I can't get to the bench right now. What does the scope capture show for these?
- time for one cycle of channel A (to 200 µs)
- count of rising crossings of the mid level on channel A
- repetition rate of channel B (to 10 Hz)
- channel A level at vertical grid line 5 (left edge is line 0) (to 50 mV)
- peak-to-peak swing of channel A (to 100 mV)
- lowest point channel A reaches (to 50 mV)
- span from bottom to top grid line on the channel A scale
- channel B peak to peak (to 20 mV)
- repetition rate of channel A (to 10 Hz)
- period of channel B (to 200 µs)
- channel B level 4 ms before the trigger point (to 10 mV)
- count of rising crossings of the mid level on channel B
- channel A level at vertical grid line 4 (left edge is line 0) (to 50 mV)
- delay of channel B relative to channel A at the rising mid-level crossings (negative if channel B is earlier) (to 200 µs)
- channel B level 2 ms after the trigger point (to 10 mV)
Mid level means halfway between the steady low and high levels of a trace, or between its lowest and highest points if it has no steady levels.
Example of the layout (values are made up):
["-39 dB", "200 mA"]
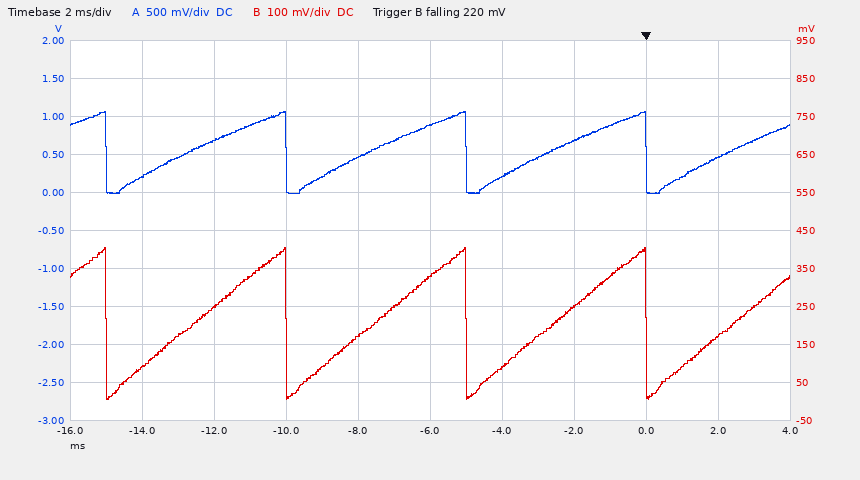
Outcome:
["5.0 ms", "4", "200 Hz", "900 mV", "1.10 V", "0 mV", "5 V", "400 mV", "200 Hz", "5.0 ms", "90 mV", "4", "450 mV", "+200 µs", "170 mV"]
